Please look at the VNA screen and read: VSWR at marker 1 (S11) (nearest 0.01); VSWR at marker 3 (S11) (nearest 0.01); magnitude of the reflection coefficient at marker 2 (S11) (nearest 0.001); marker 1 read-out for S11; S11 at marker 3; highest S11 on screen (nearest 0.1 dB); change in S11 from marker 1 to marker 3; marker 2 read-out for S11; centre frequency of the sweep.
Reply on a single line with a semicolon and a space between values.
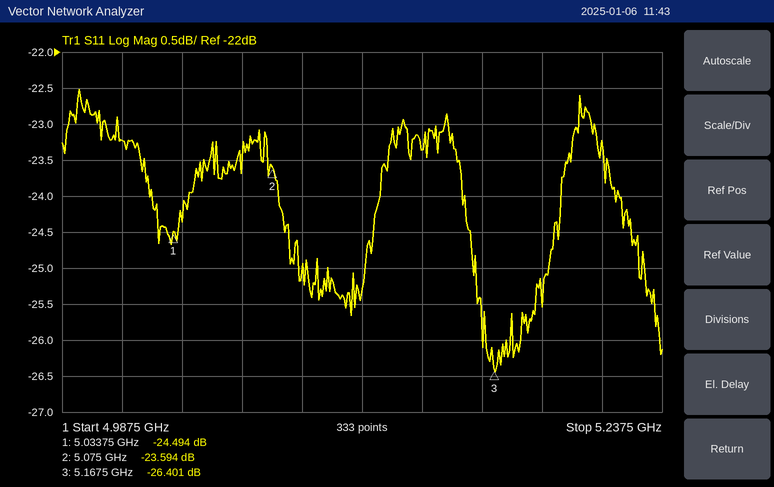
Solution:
1.13; 1.10; 0.066; -24.494 dB; -26.401 dB; -22.5 dB; -1.907 dB; -23.594 dB; 5.1125 GHz
